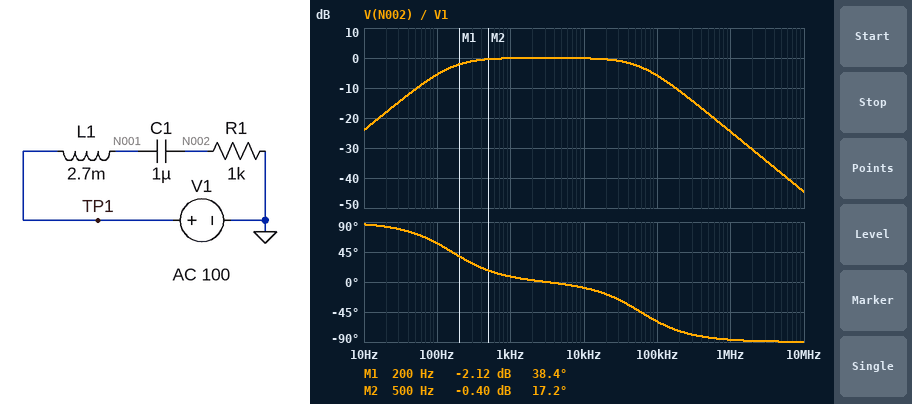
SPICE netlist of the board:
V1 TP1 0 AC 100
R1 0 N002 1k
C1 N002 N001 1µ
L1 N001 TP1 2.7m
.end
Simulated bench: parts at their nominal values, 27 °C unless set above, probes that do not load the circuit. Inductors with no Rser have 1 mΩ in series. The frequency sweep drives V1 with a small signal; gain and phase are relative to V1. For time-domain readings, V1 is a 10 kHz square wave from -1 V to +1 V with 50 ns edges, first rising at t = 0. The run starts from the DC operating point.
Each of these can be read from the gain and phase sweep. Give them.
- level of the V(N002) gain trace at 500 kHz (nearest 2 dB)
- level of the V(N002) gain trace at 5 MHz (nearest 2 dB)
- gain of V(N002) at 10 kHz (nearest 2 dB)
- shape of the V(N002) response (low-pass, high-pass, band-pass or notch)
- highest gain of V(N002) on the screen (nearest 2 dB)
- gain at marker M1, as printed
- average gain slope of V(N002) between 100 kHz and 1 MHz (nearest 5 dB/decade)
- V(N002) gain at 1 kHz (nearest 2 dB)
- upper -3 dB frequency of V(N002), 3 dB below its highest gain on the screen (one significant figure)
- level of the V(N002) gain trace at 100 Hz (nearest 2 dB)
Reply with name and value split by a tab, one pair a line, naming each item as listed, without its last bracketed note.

level of the V(N002) gain trace at 500 kHz	-18 dB
level of the V(N002) gain trace at 5 MHz	-38 dB
gain of V(N002) at 10 kHz	0 dB
shape of the V(N002) response	band-pass
highest gain of V(N002) on the screen	0 dB
gain at marker M1, as printed	-2.12 dB
average gain slope of V(N002) between 100 kHz and 1 MHz	-20 dB/decade
V(N002) gain at 1 kHz	0 dB
upper -3 dB frequency of V(N002), 3 dB below its highest gain on the screen	60 kHz
level of the V(N002) gain trace at 100 Hz	-6 dB
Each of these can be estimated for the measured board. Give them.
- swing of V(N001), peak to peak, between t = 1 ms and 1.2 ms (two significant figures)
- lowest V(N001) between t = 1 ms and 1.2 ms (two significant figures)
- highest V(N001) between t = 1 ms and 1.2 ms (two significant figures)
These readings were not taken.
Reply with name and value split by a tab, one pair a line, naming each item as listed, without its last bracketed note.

swing of V(N001), peak to peak, between t = 1 ms and 1.2 ms	2.0 V
lowest V(N001) between t = 1 ms and 1.2 ms	-1.0 V
highest V(N001) between t = 1 ms and 1.2 ms	1.0 V
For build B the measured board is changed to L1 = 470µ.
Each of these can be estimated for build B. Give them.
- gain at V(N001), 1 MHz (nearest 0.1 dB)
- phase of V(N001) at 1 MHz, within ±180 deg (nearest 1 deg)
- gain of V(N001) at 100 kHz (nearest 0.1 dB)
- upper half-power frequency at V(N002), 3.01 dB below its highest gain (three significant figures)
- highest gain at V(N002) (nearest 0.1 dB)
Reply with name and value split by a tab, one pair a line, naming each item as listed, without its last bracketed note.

gain at V(N001), 1 MHz	-9.9 dB
phase of V(N001) at 1 MHz, within ±180 deg	-71 deg
gain of V(N001) at 100 kHz	-0.4 dB
upper half-power frequency at V(N002), 3.01 dB below its highest gain	339 kHz
highest gain at V(N002)	0 dB
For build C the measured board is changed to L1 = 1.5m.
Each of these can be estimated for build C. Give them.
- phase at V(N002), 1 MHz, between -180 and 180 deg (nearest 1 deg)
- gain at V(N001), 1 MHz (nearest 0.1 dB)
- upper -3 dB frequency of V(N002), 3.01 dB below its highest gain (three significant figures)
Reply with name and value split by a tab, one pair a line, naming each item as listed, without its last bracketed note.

phase at V(N002), 1 MHz, between -180 and 180 deg	-84 deg
gain at V(N001), 1 MHz	-19.5 dB
upper -3 dB frequency of V(N002), 3.01 dB below its highest gain	106 kHz
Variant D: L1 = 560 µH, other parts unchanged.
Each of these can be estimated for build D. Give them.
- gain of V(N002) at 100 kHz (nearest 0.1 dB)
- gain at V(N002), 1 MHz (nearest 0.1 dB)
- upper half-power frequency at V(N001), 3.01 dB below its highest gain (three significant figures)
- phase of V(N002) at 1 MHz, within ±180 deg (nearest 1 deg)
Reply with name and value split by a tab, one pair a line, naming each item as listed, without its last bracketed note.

gain of V(N002) at 100 kHz	-0.5 dB
gain at V(N002), 1 MHz	-11.3 dB
upper half-power frequency at V(N001), 3.01 dB below its highest gain	284 kHz
phase of V(N002) at 1 MHz, within ±180 deg	-74 deg
